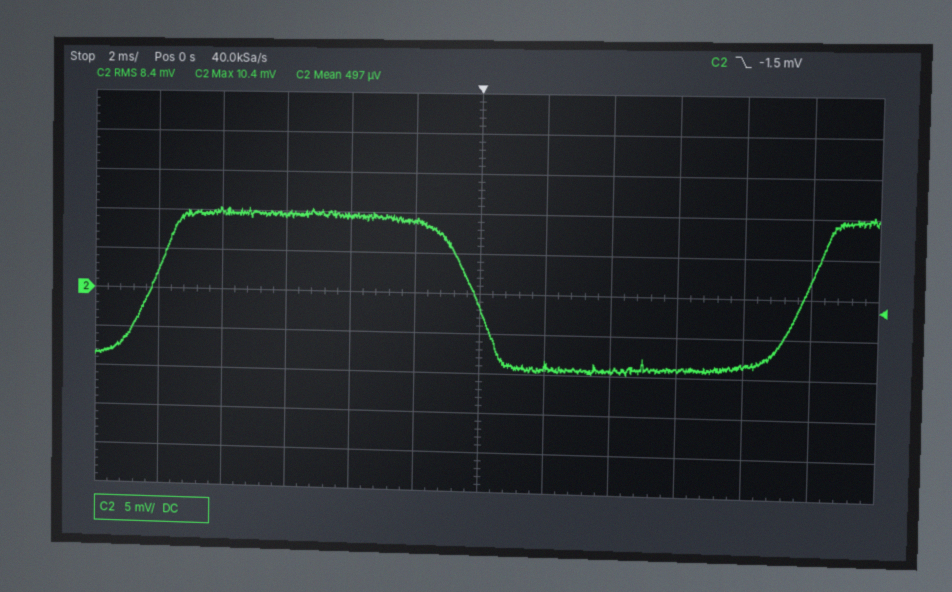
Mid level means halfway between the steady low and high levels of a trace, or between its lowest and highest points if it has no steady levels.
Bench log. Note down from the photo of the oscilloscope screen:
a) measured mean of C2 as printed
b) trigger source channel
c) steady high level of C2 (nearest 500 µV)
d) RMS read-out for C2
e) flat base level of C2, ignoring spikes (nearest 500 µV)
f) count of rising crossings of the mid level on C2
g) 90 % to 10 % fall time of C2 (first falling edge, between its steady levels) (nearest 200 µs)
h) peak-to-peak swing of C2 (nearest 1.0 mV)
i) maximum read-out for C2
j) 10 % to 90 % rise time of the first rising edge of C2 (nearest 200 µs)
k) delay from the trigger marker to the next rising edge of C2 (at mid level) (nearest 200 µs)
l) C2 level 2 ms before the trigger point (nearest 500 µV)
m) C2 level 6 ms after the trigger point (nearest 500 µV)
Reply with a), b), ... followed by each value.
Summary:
a) 497 µV
b) C2
c) 9.5 mV
d) 8.4 mV
e) -9.0 mV
f) 2
g) 1.8 ms
h) 20.0 mV
i) 10.4 mV
j) 1.8 ms
k) 9.8 ms
l) 9.0 mV
m) -9.0 mV
